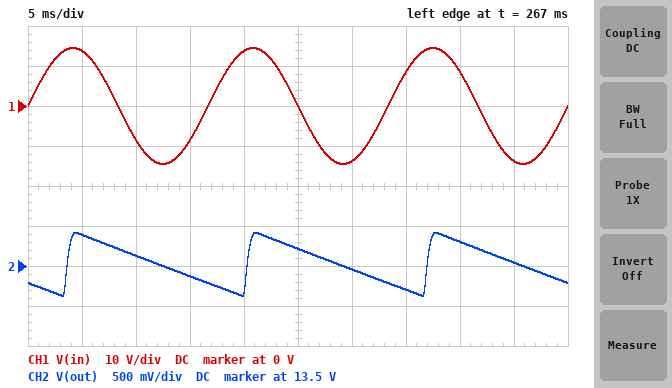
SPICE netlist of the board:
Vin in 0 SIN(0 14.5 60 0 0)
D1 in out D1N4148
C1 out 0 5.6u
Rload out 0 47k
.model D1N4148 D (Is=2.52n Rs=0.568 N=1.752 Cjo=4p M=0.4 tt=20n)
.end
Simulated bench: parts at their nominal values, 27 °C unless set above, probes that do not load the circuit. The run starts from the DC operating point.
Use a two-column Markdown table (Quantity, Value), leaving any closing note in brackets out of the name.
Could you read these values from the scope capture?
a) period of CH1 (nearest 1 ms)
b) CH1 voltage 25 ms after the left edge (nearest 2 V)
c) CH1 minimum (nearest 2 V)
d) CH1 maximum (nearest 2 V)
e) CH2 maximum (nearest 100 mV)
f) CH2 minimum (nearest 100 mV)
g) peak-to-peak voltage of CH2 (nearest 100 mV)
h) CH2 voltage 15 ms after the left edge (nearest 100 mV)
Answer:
| Quantity | Value |
|---|---|
| period of CH1 | 17 ms |
| CH1 voltage 25 ms after the left edge | 0 V |
| CH1 minimum | -14 V |
| CH1 maximum | 14 V |
| CH2 maximum | 13.9 V |
| CH2 minimum | 13.1 V |
| peak-to-peak voltage of CH2 | 800 mV |
| CH2 voltage 15 ms after the left edge | 13.4 V |
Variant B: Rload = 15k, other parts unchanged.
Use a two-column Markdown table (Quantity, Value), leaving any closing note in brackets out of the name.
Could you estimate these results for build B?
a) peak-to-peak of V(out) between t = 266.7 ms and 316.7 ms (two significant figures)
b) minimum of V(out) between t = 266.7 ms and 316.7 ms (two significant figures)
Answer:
| Quantity | Value |
|---|---|
| peak-to-peak of V(out) between t = 266.7 ms and 316.7 ms | 2.3 V |
| minimum of V(out) between t = 266.7 ms and 316.7 ms | 12 V |
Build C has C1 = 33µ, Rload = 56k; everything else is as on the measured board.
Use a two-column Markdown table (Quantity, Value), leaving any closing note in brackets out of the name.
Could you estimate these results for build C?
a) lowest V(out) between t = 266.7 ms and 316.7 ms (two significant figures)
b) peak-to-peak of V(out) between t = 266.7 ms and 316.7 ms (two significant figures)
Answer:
| Quantity | Value |
|---|---|
| lowest V(out) between t = 266.7 ms and 316.7 ms | 14 V |
| peak-to-peak of V(out) between t = 266.7 ms and 316.7 ms | 120 mV |
